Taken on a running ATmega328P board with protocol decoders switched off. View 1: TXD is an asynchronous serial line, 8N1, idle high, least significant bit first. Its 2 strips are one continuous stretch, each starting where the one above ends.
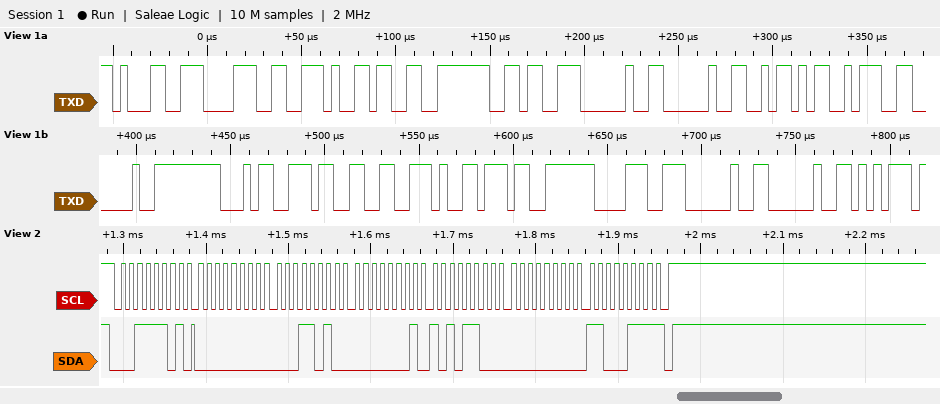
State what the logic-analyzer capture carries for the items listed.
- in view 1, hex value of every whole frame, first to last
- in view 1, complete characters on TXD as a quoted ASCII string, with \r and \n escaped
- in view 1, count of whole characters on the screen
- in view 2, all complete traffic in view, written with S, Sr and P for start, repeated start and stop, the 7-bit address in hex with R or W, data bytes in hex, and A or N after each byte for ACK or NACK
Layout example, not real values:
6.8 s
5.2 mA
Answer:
0x31 0x38 0x2E 0x33 0x36 0x20 0x20 0x5A 0x3A 0x20 0x34 0x33 0x2E 0x37 0x38 0x20 0x20 0x75
"18.36  Z: 43.78  u"
18
S 1ER A 00 A 1A A 01 A AC A 00 A C7 N P
